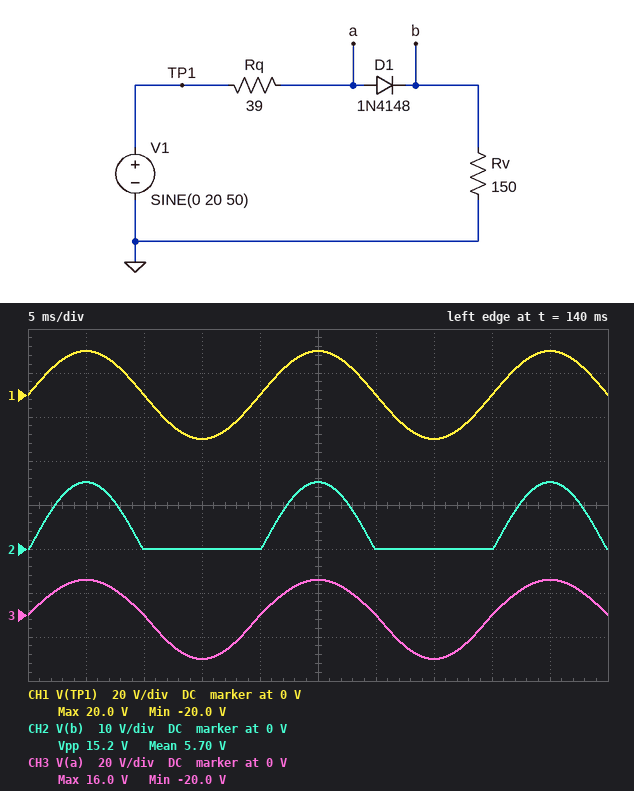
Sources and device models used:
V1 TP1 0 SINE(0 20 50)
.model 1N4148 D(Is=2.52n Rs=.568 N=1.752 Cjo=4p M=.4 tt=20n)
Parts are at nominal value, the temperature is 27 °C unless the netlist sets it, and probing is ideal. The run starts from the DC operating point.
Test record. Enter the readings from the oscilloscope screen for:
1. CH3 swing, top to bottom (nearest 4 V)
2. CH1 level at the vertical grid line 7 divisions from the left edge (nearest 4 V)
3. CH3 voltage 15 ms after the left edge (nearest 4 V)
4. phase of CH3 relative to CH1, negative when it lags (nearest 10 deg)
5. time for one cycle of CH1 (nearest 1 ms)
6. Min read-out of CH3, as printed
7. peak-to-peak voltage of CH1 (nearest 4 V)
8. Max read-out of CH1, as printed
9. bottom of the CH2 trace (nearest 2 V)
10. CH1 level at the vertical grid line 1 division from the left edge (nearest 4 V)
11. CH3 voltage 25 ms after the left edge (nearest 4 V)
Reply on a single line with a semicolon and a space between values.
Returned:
36 V; -20 V; -20 V; 0 deg; 20 ms; -20.0 V; 40 V; 20.0 V; 0 V; 20 V; 16 V
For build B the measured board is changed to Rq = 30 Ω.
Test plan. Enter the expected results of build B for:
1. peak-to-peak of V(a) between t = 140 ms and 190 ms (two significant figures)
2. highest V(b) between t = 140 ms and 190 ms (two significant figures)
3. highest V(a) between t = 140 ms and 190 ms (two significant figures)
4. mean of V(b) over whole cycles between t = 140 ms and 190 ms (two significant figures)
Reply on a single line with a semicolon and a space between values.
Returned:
37 V; 16 V; 17 V; 5.0 V
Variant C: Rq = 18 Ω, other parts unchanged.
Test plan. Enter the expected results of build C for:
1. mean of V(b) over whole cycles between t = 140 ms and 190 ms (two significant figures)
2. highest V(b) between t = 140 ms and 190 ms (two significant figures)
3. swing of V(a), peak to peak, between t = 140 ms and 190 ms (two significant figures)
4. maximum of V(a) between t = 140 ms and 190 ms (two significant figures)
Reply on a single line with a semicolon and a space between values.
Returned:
5.3 V; 17 V; 38 V; 18 V
